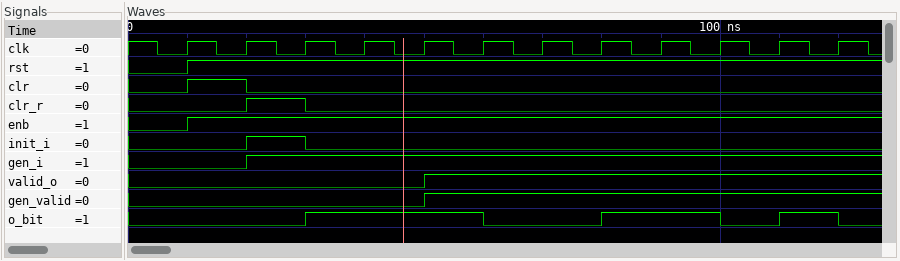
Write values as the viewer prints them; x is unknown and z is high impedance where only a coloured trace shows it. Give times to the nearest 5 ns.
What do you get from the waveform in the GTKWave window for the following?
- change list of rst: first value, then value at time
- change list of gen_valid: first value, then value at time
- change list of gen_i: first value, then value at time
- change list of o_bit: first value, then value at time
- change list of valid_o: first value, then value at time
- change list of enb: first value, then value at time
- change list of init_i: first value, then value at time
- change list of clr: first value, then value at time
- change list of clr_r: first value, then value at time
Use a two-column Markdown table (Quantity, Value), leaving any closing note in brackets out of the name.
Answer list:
| Quantity | Value |
|---|---|
| change list of rst: first value, then value at time | 0, 1 at 10 ns |
| change list of gen_valid: first value, then value at time | 0, 1 at 50 ns |
| change list of gen_i: first value, then value at time | 0, 1 at 20 ns |
| change list of o_bit: first value, then value at time | 0, 1 at 30 ns, 0 at 60 ns, 1 at 80 ns, 0 at 100 ns, 1 at 110 ns, 0 at 120 ns |
| change list of valid_o: first value, then value at time | 0, 1 at 50 ns |
| change list of enb: first value, then value at time | 0, 1 at 10 ns |
| change list of init_i: first value, then value at time | 0, 1 at 20 ns, 0 at 30 ns |
| change list of clr: first value, then value at time | 0, 1 at 10 ns, 0 at 20 ns |
| change list of clr_r: first value, then value at time | 0, 1 at 20 ns, 0 at 30 ns |
